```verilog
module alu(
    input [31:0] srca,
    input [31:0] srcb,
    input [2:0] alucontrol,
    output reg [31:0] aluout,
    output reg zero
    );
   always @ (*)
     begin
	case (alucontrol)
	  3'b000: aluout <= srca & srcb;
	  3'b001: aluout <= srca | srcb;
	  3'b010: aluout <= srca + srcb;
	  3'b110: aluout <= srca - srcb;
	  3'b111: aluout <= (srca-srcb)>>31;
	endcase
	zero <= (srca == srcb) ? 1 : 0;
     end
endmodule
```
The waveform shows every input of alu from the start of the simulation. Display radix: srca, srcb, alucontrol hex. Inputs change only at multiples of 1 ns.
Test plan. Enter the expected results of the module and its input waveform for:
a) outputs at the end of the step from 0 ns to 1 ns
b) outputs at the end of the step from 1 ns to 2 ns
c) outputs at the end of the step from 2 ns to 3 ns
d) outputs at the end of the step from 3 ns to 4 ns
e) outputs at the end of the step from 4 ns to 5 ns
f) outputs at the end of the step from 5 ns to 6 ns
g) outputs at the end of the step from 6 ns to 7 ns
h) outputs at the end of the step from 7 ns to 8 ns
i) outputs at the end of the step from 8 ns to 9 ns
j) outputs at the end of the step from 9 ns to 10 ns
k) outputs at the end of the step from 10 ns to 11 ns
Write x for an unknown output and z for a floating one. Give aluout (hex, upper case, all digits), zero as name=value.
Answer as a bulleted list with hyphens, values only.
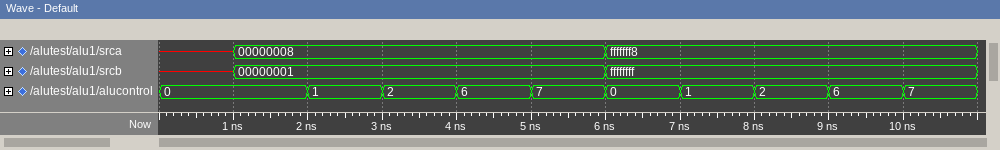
- aluout=x, zero=x
- aluout=00000000, zero=0
- aluout=00000009, zero=0
- aluout=00000009, zero=0
- aluout=00000007, zero=0
- aluout=00000000, zero=0
- aluout=FFFFFFF8, zero=0
- aluout=FFFFFFFF, zero=0
- aluout=FFFFFFF7, zero=0
- aluout=FFFFFFF9, zero=0
- aluout=00000001, zero=0
